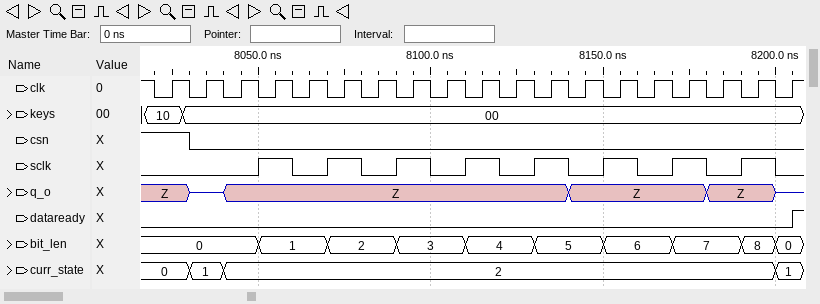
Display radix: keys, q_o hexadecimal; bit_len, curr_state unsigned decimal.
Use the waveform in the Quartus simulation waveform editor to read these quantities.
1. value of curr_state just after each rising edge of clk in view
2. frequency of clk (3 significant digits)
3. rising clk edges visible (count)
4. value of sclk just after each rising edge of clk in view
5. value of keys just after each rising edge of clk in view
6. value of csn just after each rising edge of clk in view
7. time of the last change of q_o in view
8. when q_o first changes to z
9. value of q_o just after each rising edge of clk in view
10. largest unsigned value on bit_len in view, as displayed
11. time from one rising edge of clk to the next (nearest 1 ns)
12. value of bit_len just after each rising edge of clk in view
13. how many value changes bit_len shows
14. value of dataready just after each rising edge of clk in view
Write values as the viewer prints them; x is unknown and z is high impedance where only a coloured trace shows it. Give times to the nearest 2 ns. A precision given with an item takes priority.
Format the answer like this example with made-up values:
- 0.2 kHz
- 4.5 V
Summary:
- 0, 1, 2, 2, 2, 2, 2, 2, 2, 2, 2, 2, 2, 2, 2, 2, 2, 2, 1
- 100 MHz
- 19
- 0 0 0 1 0 1 0 1 0 1 0 1 0 1 0 1 0 1 0
- 10, 00, 00, 00, 00, 00, 00, 00, 00, 00, 00, 00, 00, 00, 00, 00, 00, 00, 00
- 1 0 0 0 0 0 0 0 0 0 0 0 0 0 0 0 0 0 0
- 8200 ns
- 8030 ns
- Z, z, Z, Z, Z, Z, Z, Z, Z, Z, Z, Z, Z, Z, Z, Z, Z, Z, z
- 8
- 10 ns
- 0, 0, 0, 1, 1, 2, 2, 3, 3, 4, 4, 5, 5, 6, 6, 7, 7, 8, 0
- 9
- 0 0 0 0 0 0 0 0 0 0 0 0 0 0 0 0 0 0 1
